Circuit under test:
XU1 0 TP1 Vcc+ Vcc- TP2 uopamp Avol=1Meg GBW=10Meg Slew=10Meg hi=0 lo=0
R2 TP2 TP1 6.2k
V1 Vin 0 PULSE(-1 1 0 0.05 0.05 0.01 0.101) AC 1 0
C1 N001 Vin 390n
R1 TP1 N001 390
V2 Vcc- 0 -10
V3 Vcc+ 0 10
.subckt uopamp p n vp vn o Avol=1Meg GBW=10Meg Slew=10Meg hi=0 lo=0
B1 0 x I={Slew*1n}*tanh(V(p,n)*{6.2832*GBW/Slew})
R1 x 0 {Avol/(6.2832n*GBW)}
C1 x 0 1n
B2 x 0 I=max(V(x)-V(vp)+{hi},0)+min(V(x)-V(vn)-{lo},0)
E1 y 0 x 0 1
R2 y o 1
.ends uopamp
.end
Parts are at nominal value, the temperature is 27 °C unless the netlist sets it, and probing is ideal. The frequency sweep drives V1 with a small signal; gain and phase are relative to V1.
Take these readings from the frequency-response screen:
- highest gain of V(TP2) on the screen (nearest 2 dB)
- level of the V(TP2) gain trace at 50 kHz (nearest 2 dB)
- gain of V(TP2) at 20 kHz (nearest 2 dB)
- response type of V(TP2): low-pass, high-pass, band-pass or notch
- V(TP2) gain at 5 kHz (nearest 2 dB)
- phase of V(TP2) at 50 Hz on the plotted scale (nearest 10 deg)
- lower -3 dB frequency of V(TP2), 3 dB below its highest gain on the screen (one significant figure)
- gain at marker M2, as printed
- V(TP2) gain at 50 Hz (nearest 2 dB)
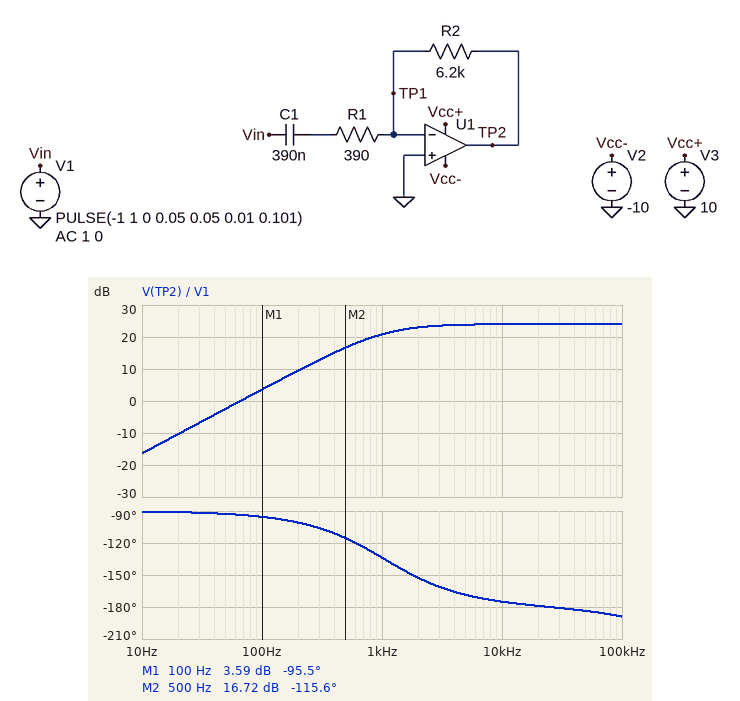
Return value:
24 dB
24 dB
24 dB
high-pass
24 dB
-90 deg
1 kHz
16.72 dB
-2 dB
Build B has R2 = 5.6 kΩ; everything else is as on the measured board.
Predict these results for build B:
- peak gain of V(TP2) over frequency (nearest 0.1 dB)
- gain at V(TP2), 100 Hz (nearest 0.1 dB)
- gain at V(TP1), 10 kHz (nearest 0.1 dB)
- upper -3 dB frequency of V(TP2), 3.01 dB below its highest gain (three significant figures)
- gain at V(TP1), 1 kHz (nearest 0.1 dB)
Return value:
23.1 dB
2.7 dB
-36.9 dB
652 kHz
-60.1 dB
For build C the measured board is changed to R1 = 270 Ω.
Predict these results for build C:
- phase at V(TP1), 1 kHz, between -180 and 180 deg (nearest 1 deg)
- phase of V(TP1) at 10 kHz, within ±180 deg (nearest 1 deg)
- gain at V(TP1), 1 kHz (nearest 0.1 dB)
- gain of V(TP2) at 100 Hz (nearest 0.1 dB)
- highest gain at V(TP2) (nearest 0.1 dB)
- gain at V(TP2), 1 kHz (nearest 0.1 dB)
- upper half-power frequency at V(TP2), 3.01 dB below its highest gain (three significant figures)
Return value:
146 deg
97 deg
-57.9 dB
3.6 dB
27.2 dB
22.1 dB
419 kHz
